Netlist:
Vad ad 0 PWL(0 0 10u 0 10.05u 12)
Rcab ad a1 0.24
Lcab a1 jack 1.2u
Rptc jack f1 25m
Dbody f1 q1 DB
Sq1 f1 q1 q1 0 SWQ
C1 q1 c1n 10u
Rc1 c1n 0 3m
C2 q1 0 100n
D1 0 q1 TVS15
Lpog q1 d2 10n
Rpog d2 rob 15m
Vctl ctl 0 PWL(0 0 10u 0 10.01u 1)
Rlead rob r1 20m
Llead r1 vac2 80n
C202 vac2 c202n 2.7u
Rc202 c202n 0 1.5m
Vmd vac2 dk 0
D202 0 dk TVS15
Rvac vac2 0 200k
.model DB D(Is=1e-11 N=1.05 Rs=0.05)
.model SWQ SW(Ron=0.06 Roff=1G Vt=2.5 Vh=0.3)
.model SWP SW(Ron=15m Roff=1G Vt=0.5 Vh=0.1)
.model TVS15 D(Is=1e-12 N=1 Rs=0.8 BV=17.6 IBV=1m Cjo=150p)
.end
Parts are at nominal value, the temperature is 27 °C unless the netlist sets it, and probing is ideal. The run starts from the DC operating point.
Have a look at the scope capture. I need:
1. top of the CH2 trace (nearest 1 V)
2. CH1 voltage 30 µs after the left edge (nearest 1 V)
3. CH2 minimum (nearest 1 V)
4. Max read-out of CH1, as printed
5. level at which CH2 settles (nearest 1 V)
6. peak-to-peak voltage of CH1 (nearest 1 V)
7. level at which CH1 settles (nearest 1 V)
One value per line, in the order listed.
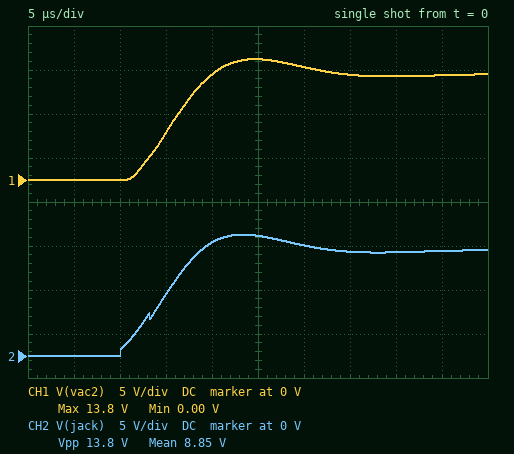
14 V
13 V
0 V
13.8 V
12 V
14 V
12 V
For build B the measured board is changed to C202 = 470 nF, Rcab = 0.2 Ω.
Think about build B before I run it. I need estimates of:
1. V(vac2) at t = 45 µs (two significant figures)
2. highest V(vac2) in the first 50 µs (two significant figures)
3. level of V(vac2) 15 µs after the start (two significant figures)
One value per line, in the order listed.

12 V
15 V
6.8 V
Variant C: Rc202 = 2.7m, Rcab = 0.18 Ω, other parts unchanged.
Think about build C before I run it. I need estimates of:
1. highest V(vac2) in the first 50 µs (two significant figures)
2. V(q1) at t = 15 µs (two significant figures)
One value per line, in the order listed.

15 V
5.9 V
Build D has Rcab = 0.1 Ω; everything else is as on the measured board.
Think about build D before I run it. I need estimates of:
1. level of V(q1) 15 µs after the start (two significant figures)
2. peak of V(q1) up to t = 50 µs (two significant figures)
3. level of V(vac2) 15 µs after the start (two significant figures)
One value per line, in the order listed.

6.5 V
17 V
6.3 V
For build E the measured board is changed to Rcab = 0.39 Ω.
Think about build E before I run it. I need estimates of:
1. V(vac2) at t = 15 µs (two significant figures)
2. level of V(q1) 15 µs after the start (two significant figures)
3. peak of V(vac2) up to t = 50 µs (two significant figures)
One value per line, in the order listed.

4.6 V
4.7 V
12 V
